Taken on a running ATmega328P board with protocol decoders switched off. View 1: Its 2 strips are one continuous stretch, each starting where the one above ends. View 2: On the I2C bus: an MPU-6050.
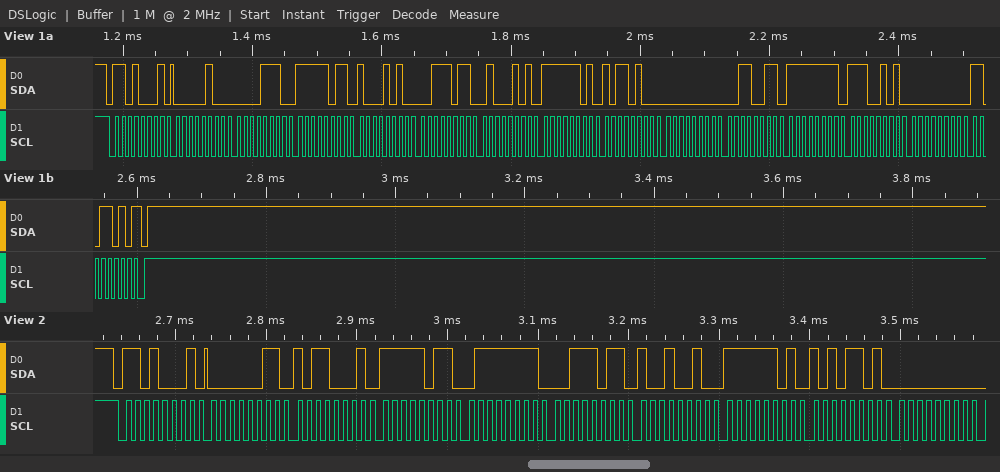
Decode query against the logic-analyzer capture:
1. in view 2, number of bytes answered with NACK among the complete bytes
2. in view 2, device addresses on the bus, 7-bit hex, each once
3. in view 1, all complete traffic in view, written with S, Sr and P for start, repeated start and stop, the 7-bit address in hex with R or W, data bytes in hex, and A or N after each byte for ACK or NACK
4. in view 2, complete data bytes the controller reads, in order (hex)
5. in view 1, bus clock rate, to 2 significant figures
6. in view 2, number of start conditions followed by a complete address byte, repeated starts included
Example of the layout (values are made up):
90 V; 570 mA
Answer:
0; 0x68; S 68R A 04 A 0E A FB A 8A A 3B A 45 A FD A B4 A 00 A 33 A FF A E5 A 00 A DA N P; 03 B1 FB 7F 3B 92 FD AD 00; 100 kHz; 1
